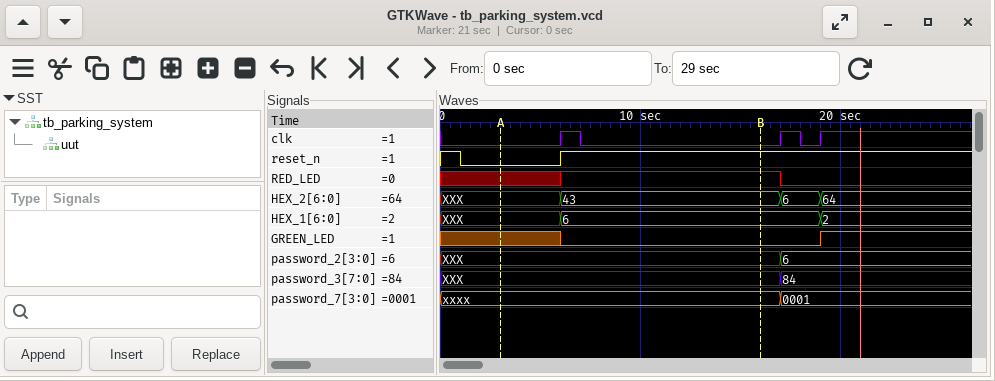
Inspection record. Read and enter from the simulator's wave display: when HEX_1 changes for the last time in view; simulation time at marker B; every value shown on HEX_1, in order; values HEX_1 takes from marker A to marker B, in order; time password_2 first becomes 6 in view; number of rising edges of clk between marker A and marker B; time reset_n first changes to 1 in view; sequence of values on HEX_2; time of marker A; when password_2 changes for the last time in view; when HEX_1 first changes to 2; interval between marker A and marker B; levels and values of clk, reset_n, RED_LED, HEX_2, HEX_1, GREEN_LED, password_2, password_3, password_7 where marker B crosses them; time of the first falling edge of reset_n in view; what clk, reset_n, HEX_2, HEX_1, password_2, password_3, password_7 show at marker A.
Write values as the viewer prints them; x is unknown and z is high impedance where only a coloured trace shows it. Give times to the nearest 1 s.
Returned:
19 s
16 s
XXX, 6, 2
XXX, 6
17 s
1
6 s
XXX, 43, 6, 64
3 s
17 s
19 s
13 s
clk=0, reset_n=1, RED_LED=1, HEX_2=43, HEX_1=6, GREEN_LED=0, password_2=XXX, password_3=XXX, password_7=xxxx
1 s
clk=0, reset_n=0, HEX_2=XXX, HEX_1=XXX, password_2=XXX, password_3=XXX, password_7=xxxx
